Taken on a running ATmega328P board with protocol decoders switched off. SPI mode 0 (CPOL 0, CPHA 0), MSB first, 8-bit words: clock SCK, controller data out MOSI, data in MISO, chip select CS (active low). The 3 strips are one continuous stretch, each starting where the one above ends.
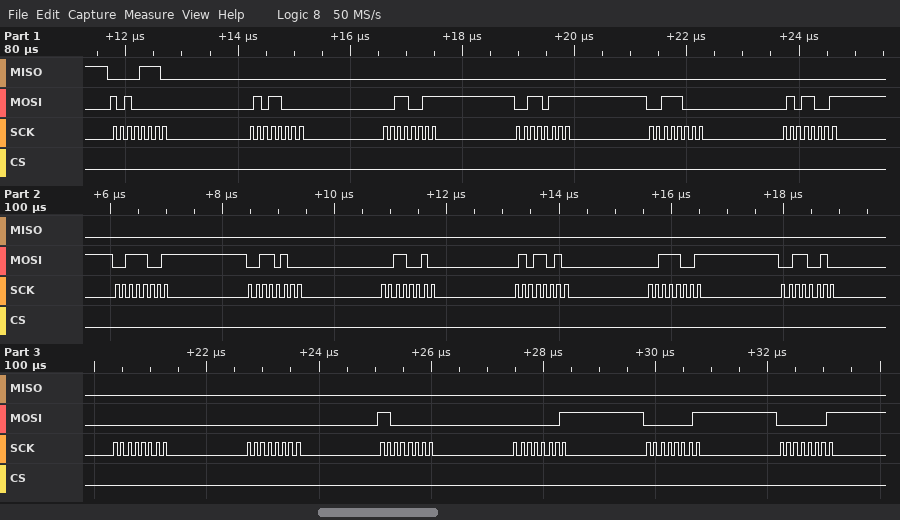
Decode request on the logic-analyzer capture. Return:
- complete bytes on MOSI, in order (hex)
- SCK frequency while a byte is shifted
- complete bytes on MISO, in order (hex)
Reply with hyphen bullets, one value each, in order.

- A0 58 33 37 38 59 39 34 32 5A 39 32 00 00 C0 01 01 01
- 8 MHz
- 0E 00 00 00 00 00 00 00 00 00 00 00 00 00 00 00 00 00
